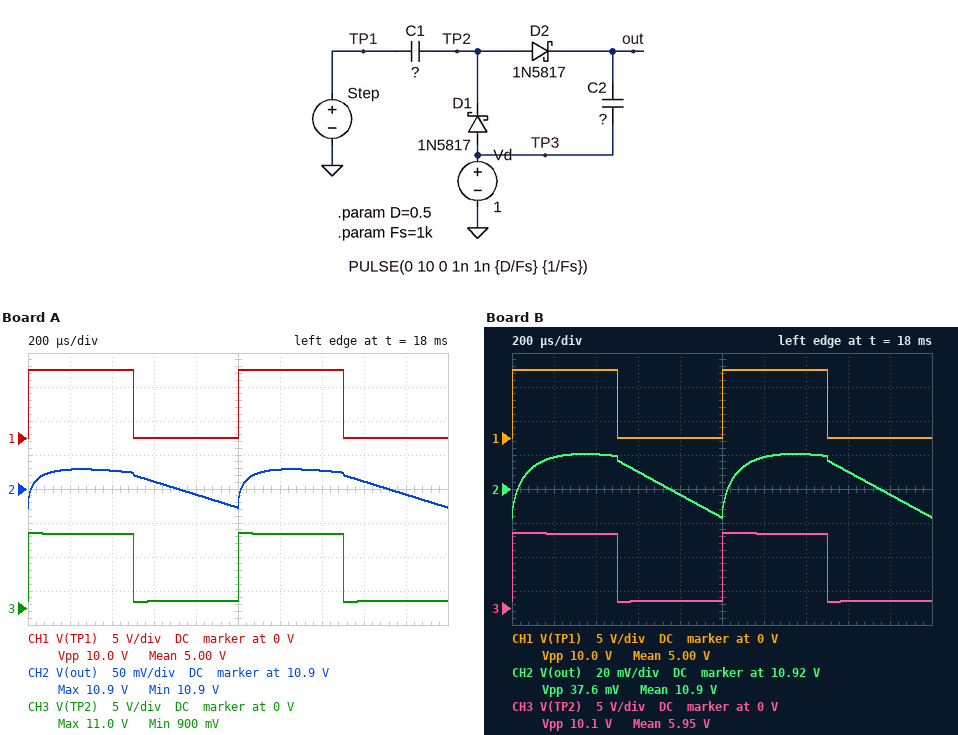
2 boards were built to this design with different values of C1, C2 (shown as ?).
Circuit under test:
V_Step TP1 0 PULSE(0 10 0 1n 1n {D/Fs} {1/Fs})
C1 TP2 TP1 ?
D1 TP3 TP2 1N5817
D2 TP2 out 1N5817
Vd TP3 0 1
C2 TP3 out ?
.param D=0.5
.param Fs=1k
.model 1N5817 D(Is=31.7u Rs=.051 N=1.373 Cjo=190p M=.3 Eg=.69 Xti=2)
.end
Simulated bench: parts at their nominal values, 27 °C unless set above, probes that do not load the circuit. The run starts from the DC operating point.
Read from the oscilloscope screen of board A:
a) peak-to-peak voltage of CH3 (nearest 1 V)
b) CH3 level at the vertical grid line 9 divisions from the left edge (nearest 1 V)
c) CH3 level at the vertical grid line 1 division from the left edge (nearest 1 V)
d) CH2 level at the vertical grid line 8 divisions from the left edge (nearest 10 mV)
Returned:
10 V
1 V
11 V
10.91 V
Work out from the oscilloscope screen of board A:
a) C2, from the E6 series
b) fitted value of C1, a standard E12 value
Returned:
330 nF
330 nF
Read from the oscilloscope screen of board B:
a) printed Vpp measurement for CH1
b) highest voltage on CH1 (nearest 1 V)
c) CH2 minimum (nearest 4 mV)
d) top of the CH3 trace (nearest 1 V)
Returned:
10.0 V
10 V
10.904 V
11 V
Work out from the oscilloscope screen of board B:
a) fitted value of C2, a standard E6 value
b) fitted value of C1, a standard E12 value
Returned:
470 nF
470 nF
